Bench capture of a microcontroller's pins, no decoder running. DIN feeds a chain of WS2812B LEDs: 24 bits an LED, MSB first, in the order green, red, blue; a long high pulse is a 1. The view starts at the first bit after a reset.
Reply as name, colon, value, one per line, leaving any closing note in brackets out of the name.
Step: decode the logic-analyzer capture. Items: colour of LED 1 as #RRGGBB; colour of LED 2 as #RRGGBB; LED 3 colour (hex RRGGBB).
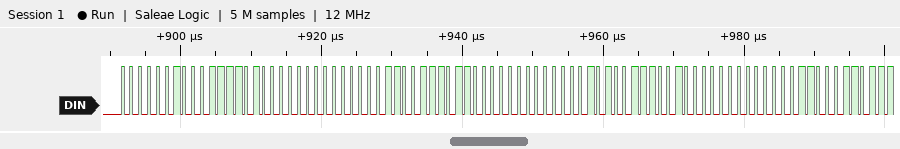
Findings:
colour of LED 1 as #RRGGBB: #3D0200
colour of LED 2 as #RRGGBB: #3B0300
LED 3 colour: #390500
